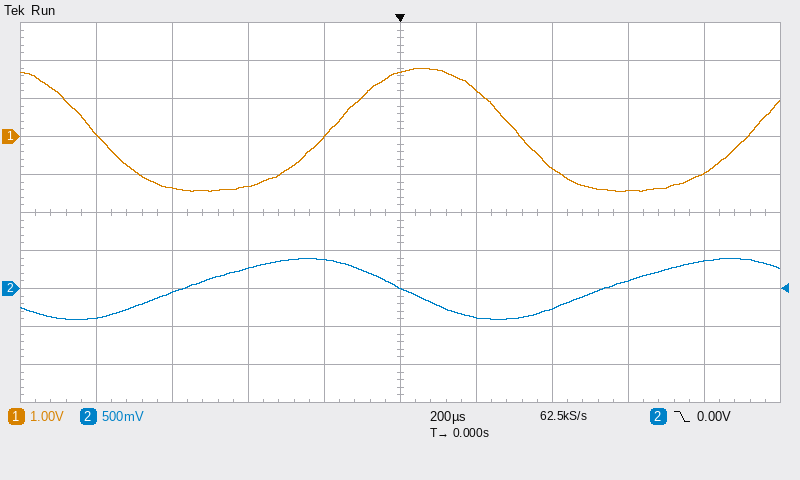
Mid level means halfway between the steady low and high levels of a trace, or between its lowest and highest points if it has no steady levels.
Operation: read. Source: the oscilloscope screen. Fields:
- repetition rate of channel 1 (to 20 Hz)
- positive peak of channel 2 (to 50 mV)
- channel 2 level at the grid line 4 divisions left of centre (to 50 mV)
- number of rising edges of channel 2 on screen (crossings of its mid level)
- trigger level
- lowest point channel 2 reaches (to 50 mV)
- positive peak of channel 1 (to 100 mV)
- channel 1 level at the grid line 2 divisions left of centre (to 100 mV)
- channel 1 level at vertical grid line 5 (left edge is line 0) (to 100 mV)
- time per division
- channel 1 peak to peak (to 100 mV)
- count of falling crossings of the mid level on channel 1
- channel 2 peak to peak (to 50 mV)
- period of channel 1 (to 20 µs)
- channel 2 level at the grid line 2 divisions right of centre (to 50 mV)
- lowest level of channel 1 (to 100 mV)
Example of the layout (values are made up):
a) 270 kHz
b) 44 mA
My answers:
a) 900 Hz
b) 400 mV
c) -400 mV
d) 2
e) 0.00 V
f) -400 mV
g) 1.8 V
h) -1.3 V
i) 1.7 V
j) 200 µs
k) 3.2 V
l) 2
m) 800 mV
n) 1.12 ms
o) -250 mV
p) -1.4 V
